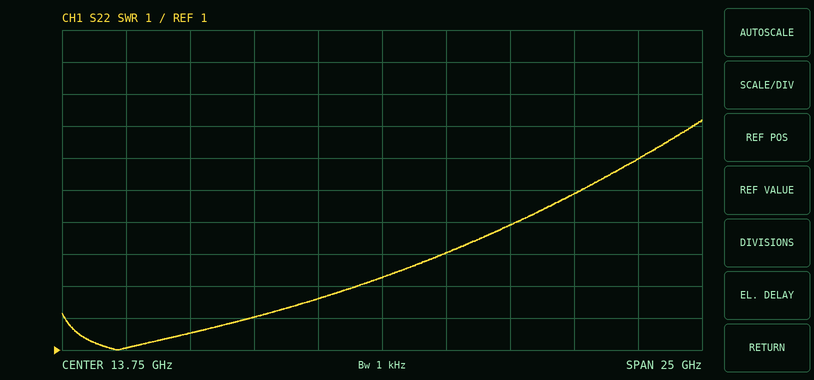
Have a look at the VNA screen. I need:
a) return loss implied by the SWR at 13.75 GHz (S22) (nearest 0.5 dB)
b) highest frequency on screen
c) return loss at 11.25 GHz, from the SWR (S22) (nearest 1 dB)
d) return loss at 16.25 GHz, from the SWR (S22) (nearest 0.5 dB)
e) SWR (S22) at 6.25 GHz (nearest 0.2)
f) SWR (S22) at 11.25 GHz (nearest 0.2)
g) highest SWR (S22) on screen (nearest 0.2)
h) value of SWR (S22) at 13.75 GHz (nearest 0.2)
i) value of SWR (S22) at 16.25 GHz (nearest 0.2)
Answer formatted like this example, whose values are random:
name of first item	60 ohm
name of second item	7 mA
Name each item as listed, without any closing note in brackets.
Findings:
return loss implied by the SWR at 13.75 GHz (S22)	5.5 dB
highest frequency on screen	26.25 GHz
return loss at 11.25 GHz, from the SWR (S22)	7 dB
return loss at 16.25 GHz, from the SWR (S22)	4.5 dB
SWR (S22) at 6.25 GHz	1.6
SWR (S22) at 11.25 GHz	2.6
highest SWR (S22) on screen	8.2
value of SWR (S22) at 13.75 GHz	3.2
value of SWR (S22) at 16.25 GHz	4.0
